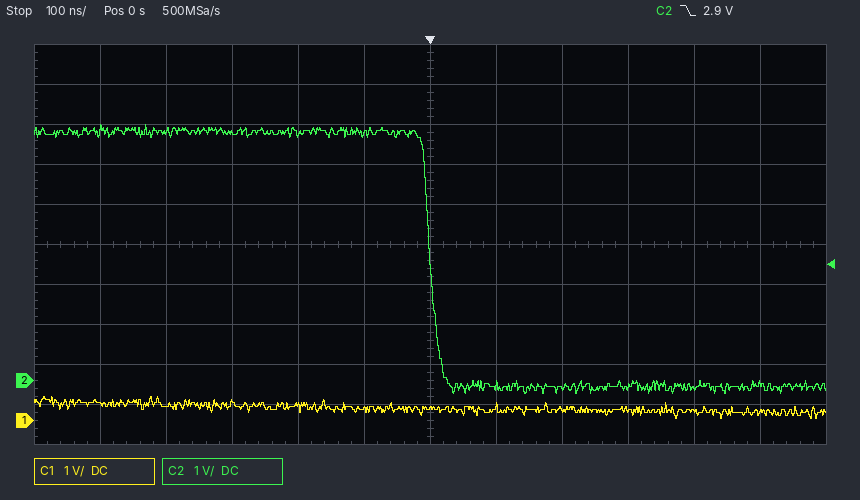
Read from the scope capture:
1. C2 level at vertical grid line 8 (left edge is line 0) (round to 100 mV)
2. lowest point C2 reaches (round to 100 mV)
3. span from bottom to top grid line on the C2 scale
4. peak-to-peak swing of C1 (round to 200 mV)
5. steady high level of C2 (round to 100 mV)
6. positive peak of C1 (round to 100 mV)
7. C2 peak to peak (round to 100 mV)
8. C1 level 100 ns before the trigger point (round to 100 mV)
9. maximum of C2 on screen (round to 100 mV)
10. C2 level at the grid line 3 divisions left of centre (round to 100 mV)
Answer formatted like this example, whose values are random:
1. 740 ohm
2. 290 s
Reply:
1. -200 mV
2. -300 mV
3. 10 V
4. 600 mV
5. 6.2 V
6. 600 mV
7. 6.7 V
8. 300 mV
9. 6.4 V
10. 6.2 V
